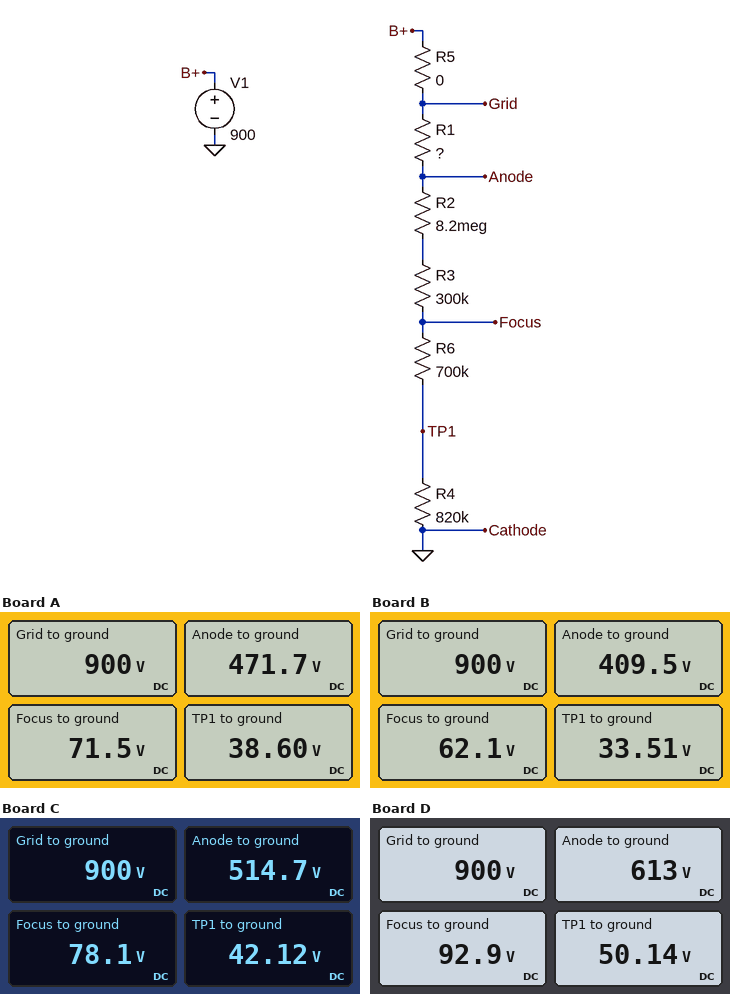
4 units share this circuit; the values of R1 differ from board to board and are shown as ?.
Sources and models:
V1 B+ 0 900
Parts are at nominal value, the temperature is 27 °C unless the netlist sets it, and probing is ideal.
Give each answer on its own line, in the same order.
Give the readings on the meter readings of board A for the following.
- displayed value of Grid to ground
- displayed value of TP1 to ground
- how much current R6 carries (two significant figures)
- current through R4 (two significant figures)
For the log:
900 V
38.60 V
47 µA
47 µA
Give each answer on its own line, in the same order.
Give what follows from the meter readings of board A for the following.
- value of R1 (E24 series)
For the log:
9.1 MΩ
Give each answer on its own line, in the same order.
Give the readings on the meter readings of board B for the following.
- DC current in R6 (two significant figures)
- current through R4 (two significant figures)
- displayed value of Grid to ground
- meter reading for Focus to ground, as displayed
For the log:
41 µA
41 µA
900 V
62.1 V
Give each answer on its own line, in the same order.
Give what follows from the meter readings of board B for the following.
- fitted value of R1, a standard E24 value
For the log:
12 MΩ
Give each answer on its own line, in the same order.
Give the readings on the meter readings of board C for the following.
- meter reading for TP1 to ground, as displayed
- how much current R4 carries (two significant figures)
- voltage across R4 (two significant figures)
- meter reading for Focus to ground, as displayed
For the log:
42.12 V
51 µA
42 V
78.1 V
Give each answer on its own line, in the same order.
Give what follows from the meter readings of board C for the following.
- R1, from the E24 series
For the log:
7.5 MΩ
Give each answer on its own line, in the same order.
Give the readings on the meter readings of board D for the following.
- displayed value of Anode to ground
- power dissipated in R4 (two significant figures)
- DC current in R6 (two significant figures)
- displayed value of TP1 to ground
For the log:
613 V
3.1 mW
61 µA
50.14 V
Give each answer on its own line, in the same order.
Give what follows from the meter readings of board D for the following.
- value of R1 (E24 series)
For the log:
4.7 MΩ
